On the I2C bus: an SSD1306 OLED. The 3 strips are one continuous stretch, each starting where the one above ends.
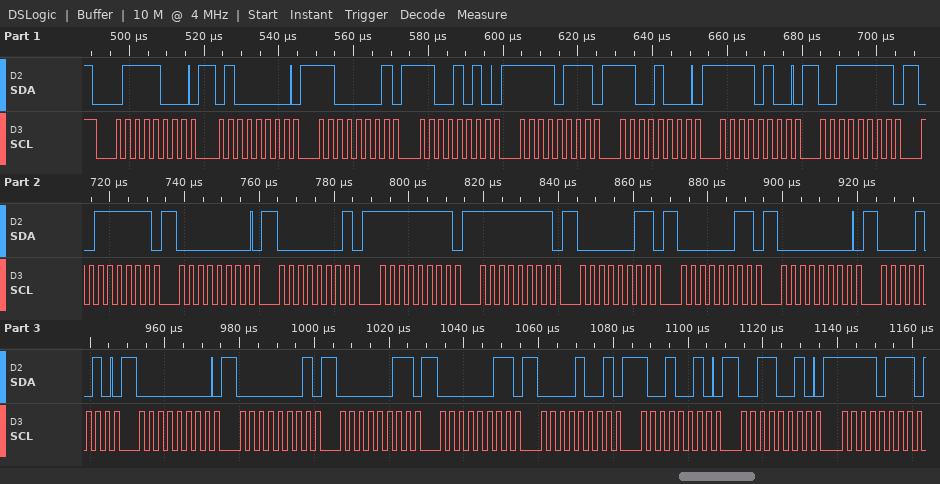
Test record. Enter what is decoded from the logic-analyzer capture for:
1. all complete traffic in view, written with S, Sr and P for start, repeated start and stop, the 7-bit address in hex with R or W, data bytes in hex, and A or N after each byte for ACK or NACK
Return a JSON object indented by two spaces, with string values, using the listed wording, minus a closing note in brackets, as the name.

{
  "all complete traffic in view, written with S, Sr and P for start, repeated start and stop, the 7-bit address in hex with R or W, data bytes in hex, and A or N after each byte for ACK or NACK": "S 3CW A 40 A C1 A CA A F7 A C8 A F4 A 3F A 3F A 00 A 01 A FF A FF A 03 A 03 A 00 A 0A A 00 A 01 A 03 A 03 A 09 A 92 A 32 A F7 A"
}
